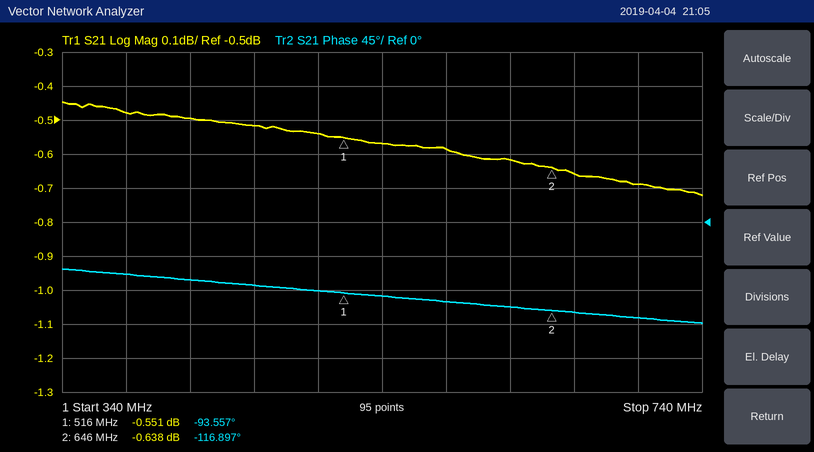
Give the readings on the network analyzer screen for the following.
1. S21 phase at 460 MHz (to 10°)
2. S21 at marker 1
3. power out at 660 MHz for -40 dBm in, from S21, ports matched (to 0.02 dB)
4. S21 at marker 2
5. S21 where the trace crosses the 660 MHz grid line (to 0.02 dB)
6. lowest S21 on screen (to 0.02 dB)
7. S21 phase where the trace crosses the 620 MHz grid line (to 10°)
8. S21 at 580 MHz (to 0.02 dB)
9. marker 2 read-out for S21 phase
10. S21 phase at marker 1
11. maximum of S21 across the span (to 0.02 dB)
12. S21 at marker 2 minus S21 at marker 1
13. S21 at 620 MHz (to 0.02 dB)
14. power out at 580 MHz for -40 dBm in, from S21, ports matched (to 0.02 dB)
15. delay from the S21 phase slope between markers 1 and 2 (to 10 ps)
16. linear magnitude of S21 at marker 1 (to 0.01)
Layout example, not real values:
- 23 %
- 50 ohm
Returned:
- -80°
- -0.551 dB
- -40.66 dBm
- -0.638 dB
- -0.66 dB
- -0.72 dB
- -110°
- -0.58 dB
- -116.897°
- -93.557°
- -0.44 dB
- -0.087 dB
- -0.62 dB
- -40.58 dBm
- 500 ps
- 0.94
